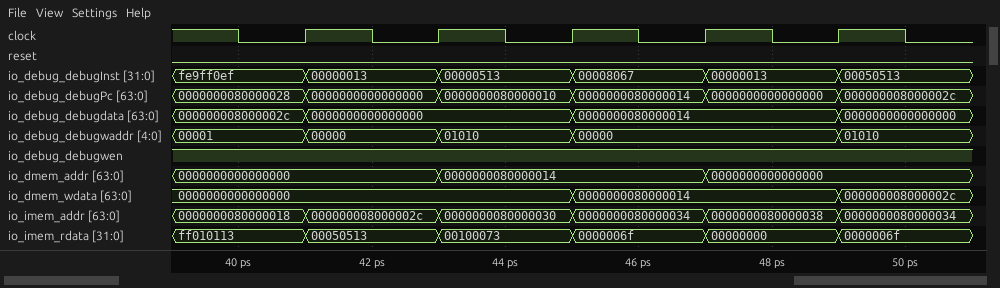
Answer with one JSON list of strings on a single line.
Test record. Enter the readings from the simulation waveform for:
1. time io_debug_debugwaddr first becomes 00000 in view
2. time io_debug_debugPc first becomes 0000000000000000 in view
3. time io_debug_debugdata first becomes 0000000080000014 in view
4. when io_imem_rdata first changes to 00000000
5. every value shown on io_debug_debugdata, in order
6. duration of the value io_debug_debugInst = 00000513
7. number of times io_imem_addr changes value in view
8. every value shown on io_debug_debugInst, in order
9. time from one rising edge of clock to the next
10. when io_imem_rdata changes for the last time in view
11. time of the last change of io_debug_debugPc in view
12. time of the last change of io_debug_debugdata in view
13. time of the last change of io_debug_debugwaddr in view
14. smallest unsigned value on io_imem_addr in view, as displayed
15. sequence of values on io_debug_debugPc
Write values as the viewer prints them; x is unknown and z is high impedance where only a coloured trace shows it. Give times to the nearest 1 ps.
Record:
["41 ps", "41 ps", "45 ps", "47 ps", "000000008000002c, 0000000000000000, 0000000080000014, 0000000000000000", "2 ps", "5", "fe9ff0ef, 00000013, 00000513, 00008067, 00000013, 00050513", "2 ps", "49 ps", "49 ps", "49 ps", "49 ps", "0000000080000018", "0000000080000028, 0000000000000000, 0000000080000010, 0000000080000014, 0000000000000000, 000000008000002c"]
